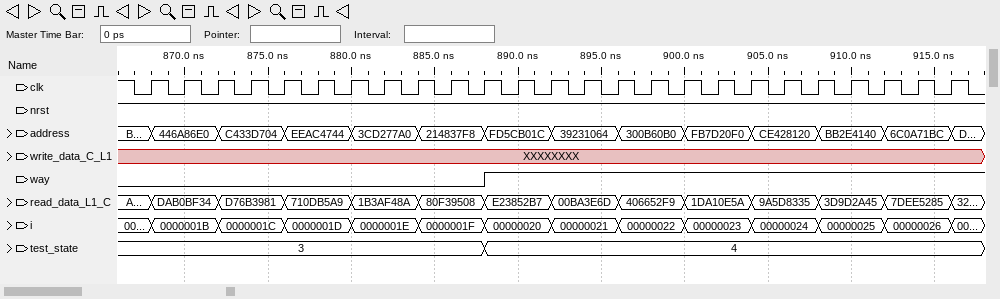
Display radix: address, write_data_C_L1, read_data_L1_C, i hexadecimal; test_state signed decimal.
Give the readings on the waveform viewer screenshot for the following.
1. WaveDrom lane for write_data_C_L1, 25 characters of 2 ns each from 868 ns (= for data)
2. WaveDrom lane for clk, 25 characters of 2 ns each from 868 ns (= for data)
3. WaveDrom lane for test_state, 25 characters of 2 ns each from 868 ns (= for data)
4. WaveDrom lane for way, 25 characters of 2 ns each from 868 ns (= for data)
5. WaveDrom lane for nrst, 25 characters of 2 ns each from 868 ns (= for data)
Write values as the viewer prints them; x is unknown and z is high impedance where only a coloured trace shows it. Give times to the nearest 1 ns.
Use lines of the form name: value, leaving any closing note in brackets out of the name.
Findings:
WaveDrom lane for write_data_C_L1, 25 characters of 2 ns each from 868 ns: {name: 'write_data_C_L1', wave: 'x........................'}
WaveDrom lane for clk, 25 characters of 2 ns each from 868 ns: {name: 'clk', wave: 'p........................'}
WaveDrom lane for test_state, 25 characters of 2 ns each from 868 ns: {name: 'test_state', wave: '=.........=..............', data: '3 4'}
WaveDrom lane for way, 25 characters of 2 ns each from 868 ns: {name: 'way', wave: '0.........1..............'}
WaveDrom lane for nrst, 25 characters of 2 ns each from 868 ns: {name: 'nrst', wave: '1........................'}
